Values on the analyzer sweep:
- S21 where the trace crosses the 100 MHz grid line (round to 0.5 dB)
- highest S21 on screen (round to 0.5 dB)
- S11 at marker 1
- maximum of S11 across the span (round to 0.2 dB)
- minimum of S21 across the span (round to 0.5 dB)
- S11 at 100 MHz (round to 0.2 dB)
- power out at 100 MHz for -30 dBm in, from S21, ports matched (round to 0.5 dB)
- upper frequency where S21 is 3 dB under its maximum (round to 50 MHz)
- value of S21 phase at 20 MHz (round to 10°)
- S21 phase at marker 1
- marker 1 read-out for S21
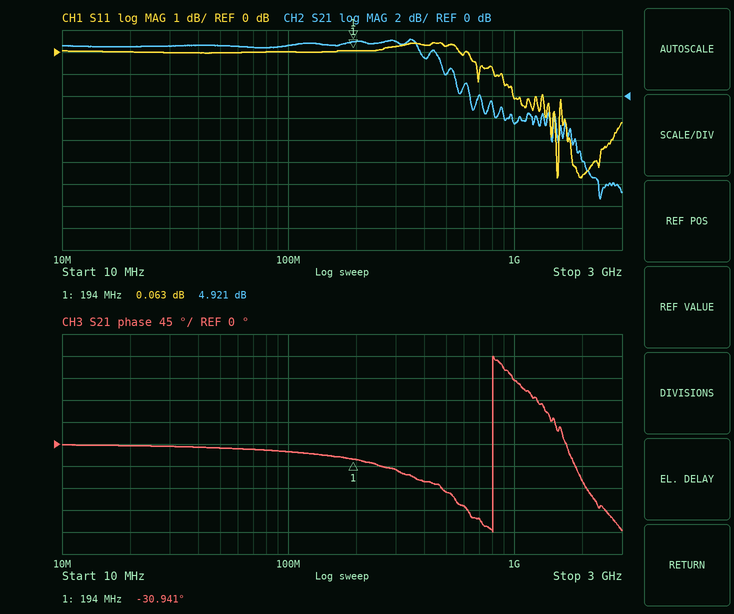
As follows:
4.5 dB
5.0 dB
0.063 dB
0.4 dB
-9.5 dB
0.0 dB
-25.5 dBm
500 MHz
0°
-30.941°
4.921 dB
